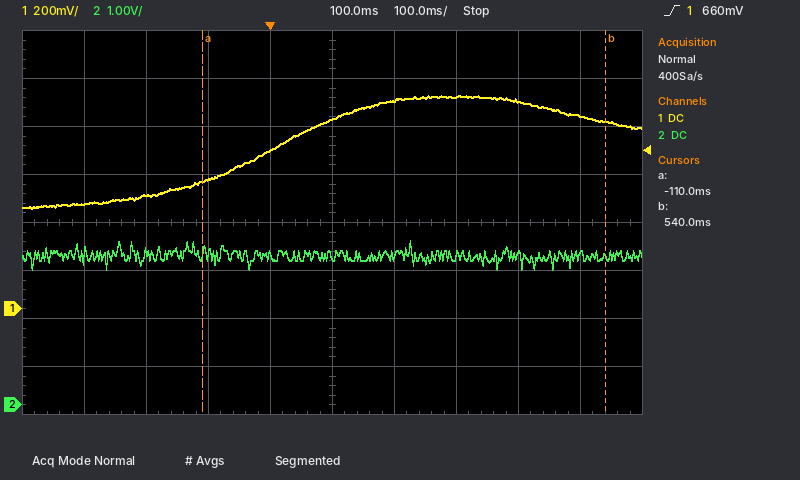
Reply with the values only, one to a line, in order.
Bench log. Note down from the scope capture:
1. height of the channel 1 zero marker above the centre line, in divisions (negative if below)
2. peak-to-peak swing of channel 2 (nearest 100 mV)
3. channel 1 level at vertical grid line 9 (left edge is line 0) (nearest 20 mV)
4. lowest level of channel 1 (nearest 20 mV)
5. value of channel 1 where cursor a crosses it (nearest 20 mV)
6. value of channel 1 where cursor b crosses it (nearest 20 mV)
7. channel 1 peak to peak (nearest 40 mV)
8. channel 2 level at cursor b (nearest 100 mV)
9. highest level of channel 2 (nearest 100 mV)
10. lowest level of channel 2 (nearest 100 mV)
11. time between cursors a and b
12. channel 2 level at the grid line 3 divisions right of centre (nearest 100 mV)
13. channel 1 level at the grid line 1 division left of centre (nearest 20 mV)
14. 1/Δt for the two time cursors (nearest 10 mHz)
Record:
-1.8 div
600 mV
800 mV
420 mV
540 mV
780 mV
480 mV
3.1 V
3.4 V
2.8 V
650 ms
3.1 V
660 mV
1.54 Hz
